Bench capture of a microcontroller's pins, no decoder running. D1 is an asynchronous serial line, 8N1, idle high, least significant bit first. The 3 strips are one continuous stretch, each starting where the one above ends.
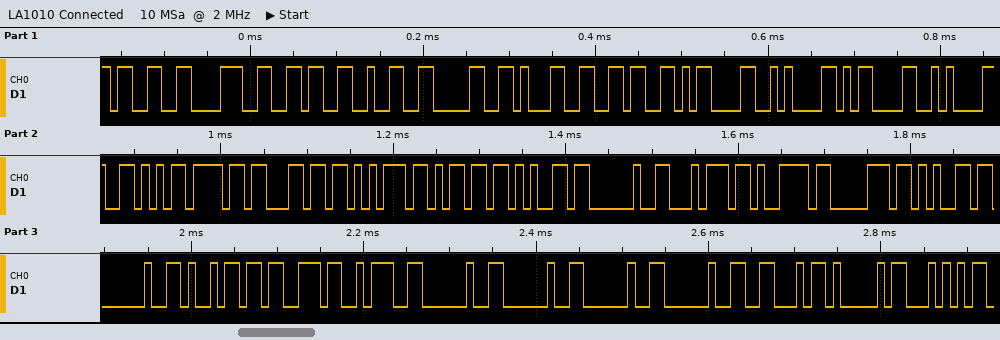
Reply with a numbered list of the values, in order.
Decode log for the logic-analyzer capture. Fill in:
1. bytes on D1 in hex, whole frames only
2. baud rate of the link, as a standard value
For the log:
1. 33 38 36 32 30 31 36 0D 0A 0D 0A 56 6F 6C 75 6D 65 20 74 79 70 65 20 69 73 3A 20 20 20 20 46 41 54
2. 115200 baud
